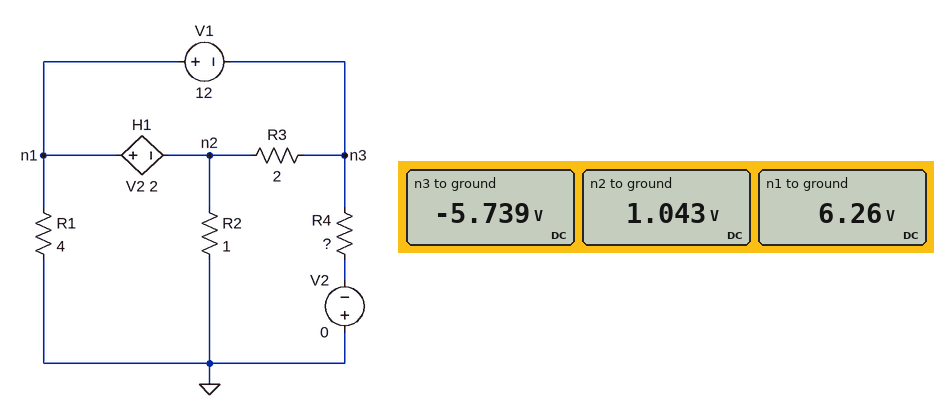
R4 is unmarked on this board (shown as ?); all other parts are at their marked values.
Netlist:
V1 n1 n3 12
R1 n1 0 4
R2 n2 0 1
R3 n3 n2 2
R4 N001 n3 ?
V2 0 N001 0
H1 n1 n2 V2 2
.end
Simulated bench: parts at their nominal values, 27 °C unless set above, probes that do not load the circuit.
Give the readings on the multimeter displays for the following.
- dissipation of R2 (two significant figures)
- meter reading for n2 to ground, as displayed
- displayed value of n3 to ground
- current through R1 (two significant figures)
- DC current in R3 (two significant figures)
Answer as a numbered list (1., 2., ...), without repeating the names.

1. 1.1 W
2. 1.043 V
3. -5.739 V
4. 1.6 A
5. 3.4 A
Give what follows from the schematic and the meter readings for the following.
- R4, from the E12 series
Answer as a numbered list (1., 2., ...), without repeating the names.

1. 2.2 Ω
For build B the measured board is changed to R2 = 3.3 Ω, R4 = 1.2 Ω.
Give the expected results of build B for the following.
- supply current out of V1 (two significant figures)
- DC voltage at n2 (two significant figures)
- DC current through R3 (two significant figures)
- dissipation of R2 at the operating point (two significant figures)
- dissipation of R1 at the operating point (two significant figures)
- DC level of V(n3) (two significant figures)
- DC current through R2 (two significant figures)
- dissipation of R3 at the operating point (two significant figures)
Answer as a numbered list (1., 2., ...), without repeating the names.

1. 6.0 A
2. 2.6 V
3. 3.1 A
4. 2.1 W
5. 18 W
6. -3.5 V
7. 800 mA
8. 19 W
